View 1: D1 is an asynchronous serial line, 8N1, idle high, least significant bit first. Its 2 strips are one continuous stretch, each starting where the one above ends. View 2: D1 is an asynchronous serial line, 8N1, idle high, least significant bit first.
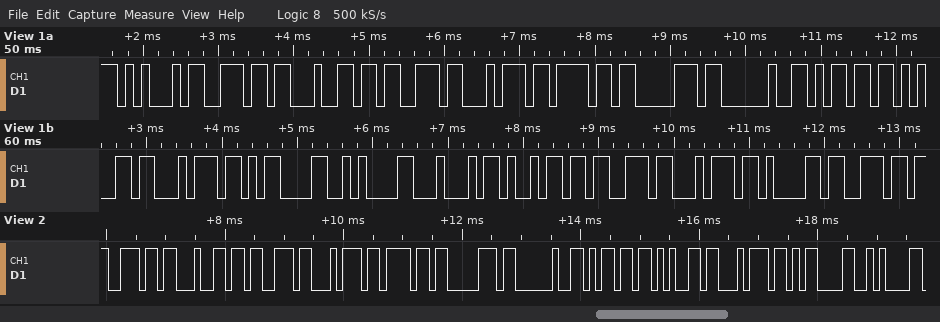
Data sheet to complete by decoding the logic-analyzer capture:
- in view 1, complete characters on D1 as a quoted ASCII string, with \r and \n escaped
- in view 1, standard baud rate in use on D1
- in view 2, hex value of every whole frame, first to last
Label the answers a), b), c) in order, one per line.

a) "Endstop met\r\nDistan"
b) 9600 baud
c) 6E 64 73 74 6F 70 20 6D 65 74 0D 0A
